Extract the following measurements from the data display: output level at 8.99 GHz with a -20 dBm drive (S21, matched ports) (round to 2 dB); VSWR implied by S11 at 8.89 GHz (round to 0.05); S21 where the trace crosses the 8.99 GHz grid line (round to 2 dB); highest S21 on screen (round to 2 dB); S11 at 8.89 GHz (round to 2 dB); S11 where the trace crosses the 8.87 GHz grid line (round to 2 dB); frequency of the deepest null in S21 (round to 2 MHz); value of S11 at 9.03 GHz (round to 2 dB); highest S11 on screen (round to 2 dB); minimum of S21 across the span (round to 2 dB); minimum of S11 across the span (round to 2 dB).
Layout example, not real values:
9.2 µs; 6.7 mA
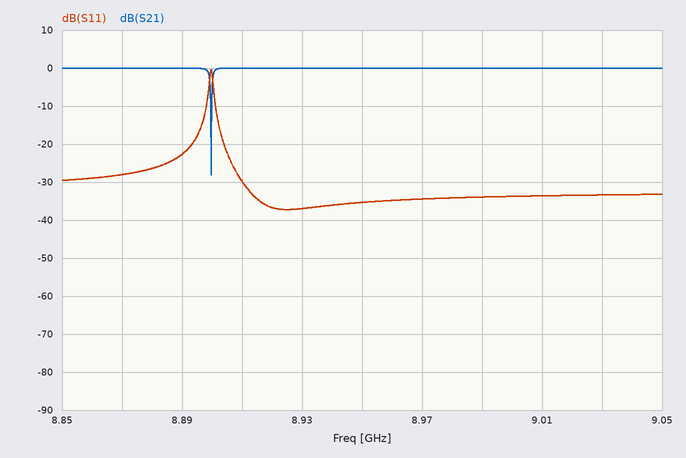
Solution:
-20 dBm; 1.15; 0 dB; 0 dB; -22 dB; -28 dB; 8.900 GHz; -34 dB; 0 dB; -28 dB; -38 dB
